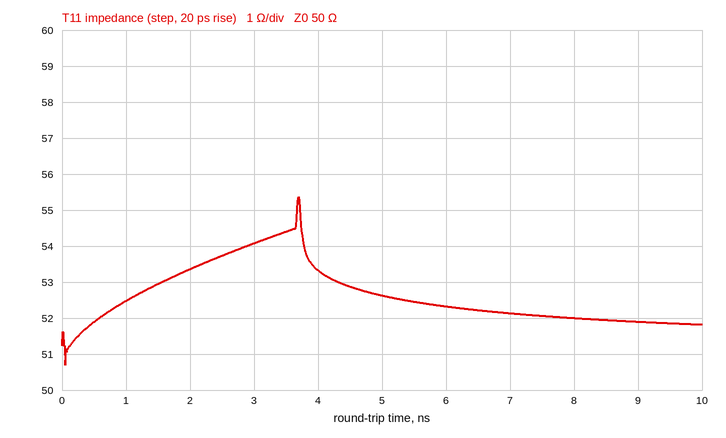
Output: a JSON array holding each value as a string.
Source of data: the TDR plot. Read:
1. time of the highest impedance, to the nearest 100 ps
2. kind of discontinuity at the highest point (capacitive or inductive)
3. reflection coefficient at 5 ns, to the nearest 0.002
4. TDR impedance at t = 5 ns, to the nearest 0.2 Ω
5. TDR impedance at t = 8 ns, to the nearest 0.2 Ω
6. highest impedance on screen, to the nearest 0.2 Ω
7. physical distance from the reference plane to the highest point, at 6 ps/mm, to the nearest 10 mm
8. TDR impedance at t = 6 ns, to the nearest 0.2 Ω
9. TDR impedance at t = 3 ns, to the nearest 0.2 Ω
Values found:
["3.7 ns", "inductive", "+0.026", "52.6 Ω", "52.0 Ω", "55.4 Ω", "310 mm", "52.4 Ω", "54.0 Ω"]
